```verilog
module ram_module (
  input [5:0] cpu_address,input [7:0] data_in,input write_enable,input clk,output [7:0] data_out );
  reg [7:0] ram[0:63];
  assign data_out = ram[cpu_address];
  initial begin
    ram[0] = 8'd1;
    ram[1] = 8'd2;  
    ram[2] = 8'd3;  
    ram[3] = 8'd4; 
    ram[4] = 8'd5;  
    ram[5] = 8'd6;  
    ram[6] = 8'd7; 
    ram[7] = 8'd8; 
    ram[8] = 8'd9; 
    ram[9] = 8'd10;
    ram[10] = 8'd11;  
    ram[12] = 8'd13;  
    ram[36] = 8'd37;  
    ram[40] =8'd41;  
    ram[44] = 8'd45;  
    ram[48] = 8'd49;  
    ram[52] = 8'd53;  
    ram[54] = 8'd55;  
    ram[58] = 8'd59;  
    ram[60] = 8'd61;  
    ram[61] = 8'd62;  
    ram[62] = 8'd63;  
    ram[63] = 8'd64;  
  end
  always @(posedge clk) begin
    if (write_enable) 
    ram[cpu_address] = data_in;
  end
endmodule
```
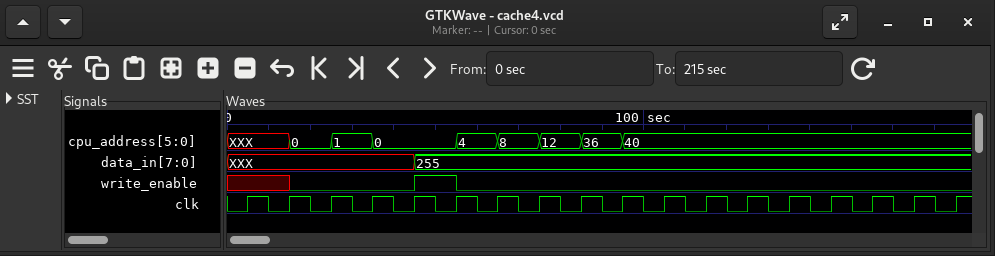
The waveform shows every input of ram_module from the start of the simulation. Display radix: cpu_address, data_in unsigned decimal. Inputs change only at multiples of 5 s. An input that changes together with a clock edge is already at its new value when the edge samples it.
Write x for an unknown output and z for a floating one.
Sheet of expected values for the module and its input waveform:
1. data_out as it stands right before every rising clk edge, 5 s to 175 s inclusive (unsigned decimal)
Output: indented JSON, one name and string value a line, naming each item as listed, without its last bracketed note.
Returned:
{
  "data_out as it stands right before every rising clk edge, 5 s to 175 s inclusive": "x, x, 1, 2, 1, 255, 5, 9, 13, 37, 41, 41, 41, 41, 41, 41, 41, 41"
}
